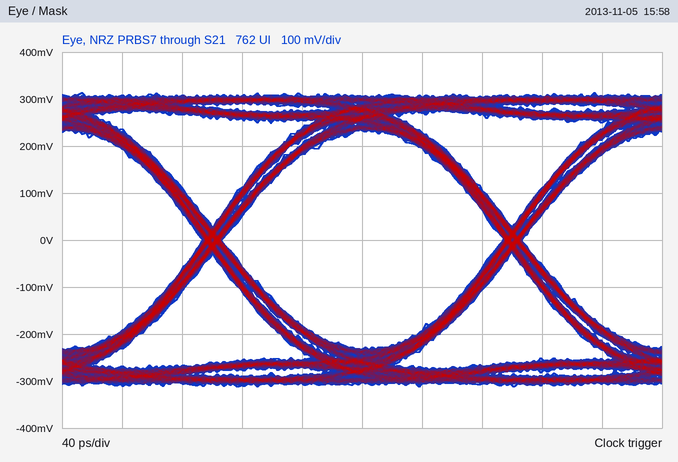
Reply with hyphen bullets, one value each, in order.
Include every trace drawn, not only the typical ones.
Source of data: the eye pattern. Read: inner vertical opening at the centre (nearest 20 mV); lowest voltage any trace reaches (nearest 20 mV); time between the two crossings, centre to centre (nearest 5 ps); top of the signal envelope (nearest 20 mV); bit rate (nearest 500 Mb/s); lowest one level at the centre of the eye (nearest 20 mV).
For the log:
- 460 mV
- -320 mV
- 200 ps
- 320 mV
- 5.0 Gb/s
- 240 mV
